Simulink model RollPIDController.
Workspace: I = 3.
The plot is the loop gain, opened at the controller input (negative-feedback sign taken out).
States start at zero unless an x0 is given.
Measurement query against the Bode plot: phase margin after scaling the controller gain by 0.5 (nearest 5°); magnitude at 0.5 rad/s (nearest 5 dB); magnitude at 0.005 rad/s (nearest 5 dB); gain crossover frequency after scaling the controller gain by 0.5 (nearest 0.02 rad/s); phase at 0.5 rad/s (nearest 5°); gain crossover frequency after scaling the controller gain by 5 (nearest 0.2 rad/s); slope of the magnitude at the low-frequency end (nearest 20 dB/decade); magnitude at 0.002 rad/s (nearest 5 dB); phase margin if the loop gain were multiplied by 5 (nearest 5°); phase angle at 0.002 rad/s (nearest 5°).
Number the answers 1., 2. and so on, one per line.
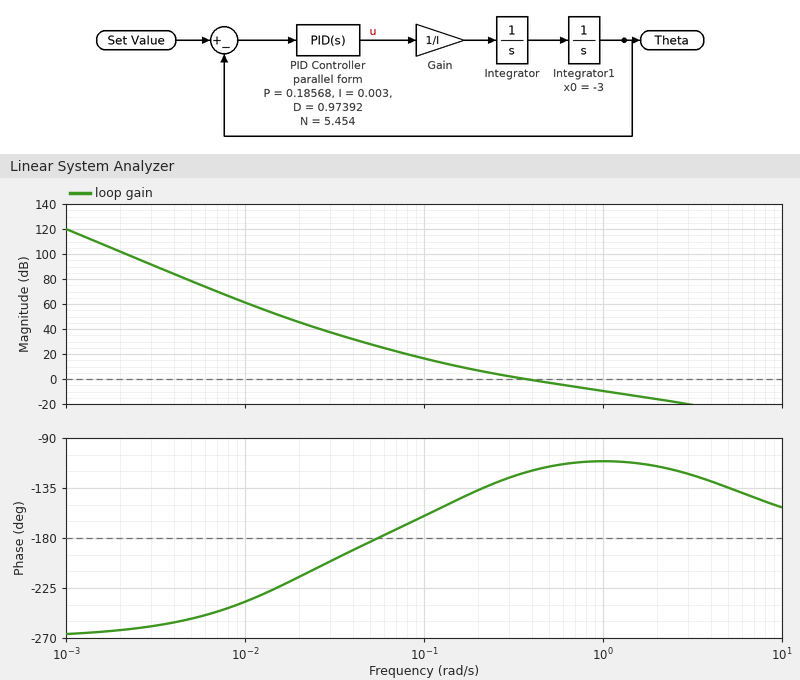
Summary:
1. 45°
2. -5 dB
3. 80 dB
4. 0.22 rad/s
5. -115°
6. 1.6 rad/s
7. -60 dB/decade
8. 100 dB
9. 65°
10. -265°
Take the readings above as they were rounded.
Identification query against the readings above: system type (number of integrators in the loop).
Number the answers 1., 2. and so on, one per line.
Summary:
1. 3
